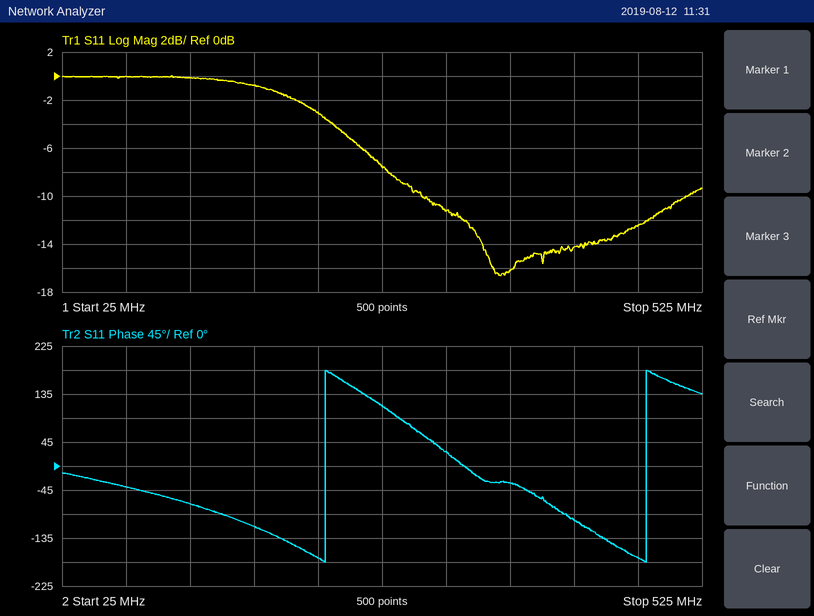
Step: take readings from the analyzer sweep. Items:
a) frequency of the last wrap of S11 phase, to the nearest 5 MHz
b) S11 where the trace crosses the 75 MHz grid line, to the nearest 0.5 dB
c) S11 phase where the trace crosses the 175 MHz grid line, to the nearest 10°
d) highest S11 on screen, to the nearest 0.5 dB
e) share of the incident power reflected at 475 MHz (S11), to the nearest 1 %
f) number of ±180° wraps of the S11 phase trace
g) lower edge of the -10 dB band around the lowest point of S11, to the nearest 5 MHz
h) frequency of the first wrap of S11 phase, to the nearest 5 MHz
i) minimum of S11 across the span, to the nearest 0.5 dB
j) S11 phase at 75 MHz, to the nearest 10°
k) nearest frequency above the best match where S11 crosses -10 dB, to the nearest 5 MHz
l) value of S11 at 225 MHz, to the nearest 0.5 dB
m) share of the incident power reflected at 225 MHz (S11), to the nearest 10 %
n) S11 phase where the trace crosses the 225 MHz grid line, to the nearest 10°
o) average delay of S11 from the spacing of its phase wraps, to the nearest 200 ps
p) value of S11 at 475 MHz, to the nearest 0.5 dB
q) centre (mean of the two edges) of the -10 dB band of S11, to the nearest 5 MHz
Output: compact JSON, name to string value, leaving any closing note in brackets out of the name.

{"frequency of the last wrap of S11 phase, to the nearest 5 MHz": "480 MHz", "S11 where the trace crosses the 75 MHz grid line, to the nearest 0.5 dB": "0.0 dB", "S11 phase where the trace crosses the 175 MHz grid line, to the nearest 10°": "-110°", "highest S11 on screen, to the nearest 0.5 dB": "0.0 dB", "share of the incident power reflected at 475 MHz (S11), to the nearest 1 %": "6 %", "number of ±180° wraps of the S11 phase trace": "2", "lower edge of the -10 dB band around the lowest point of S11, to the nearest 5 MHz": "305 MHz", "frequency of the first wrap of S11 phase, to the nearest 5 MHz": "230 MHz", "minimum of S11 across the span, to the nearest 0.5 dB": "-16.5 dB", "S11 phase at 75 MHz, to the nearest 10°": "-40°", "nearest frequency above the best match where S11 crosses -10 dB, to the nearest 5 MHz": "515 MHz", "value of S11 at 225 MHz, to the nearest 0.5 dB": "-3.0 dB", "share of the incident power reflected at 225 MHz (S11), to the nearest 10 %": "50 %", "S11 phase where the trace crosses the 225 MHz grid line, to the nearest 10°": "-170°", "average delay of S11 from the spacing of its phase wraps, to the nearest 200 ps": "4.0 ns", "value of S11 at 475 MHz, to the nearest 0.5 dB": "-12.5 dB", "centre (mean of the two edges) of the -10 dB band of S11, to the nearest 5 MHz": "410 MHz"}
